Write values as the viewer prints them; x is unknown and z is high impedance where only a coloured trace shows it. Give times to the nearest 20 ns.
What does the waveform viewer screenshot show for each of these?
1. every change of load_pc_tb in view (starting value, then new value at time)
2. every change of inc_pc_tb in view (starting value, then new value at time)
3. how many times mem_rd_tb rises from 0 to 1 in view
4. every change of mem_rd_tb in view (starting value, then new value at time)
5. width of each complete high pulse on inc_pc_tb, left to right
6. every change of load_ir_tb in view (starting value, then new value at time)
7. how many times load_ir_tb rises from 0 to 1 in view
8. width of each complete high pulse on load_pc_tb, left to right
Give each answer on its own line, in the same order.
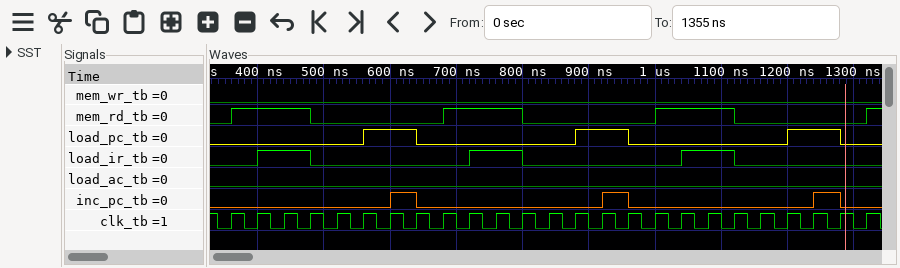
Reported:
0, 1 at 560 ns, 0 at 640 ns, 1 at 880 ns, 0 at 960 ns, 1 at 1200 ns, 0 at 1280 ns
0, 1 at 600 ns, 0 at 640 ns, 1 at 920 ns, 0 at 960 ns, 1 at 1240 ns, 0 at 1280 ns
4
0, 1 at 360 ns, 0 at 480 ns, 1 at 680 ns, 0 at 800 ns, 1 at 1000 ns, 0 at 1120 ns, 1 at 1320 ns
40 ns, 40 ns, 40 ns
0, 1 at 400 ns, 0 at 480 ns, 1 at 720 ns, 0 at 800 ns, 1 at 1040 ns, 0 at 1120 ns
3
80 ns, 80 ns, 80 ns
